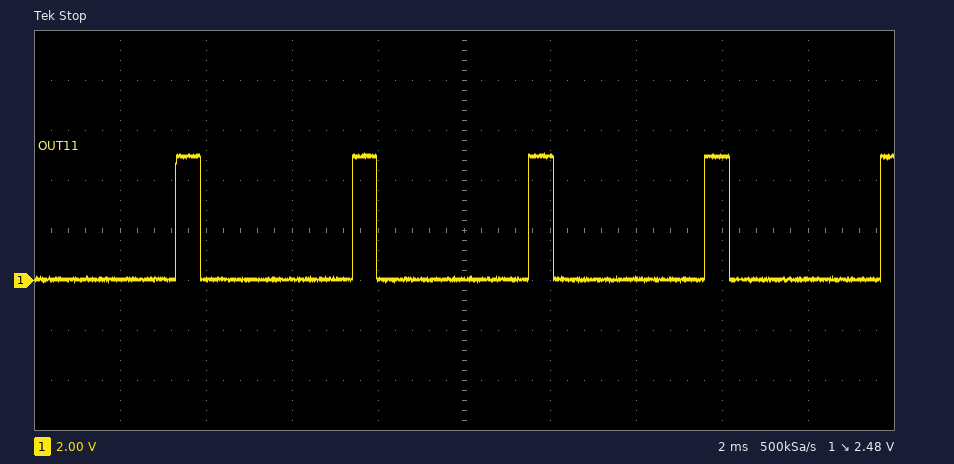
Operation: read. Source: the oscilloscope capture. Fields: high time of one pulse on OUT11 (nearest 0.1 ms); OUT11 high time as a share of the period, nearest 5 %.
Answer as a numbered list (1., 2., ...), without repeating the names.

1. 0.6 ms
2. 15 %
